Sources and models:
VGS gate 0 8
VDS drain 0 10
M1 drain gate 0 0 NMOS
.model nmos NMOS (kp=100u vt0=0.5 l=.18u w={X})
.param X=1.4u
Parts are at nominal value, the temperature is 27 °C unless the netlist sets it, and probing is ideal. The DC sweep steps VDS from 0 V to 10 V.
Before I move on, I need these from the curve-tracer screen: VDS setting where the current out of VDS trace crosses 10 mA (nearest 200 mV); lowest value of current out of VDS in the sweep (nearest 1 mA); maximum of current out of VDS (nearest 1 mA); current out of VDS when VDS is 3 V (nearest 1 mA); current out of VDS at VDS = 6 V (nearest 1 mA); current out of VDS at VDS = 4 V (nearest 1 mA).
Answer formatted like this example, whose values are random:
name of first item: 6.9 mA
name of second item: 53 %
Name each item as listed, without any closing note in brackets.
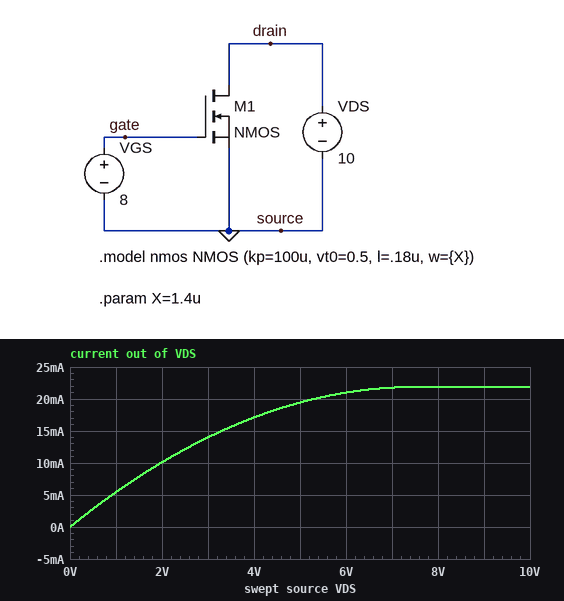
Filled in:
VDS setting where the current out of VDS trace crosses 10 mA: 2.0 V
lowest value of current out of VDS in the sweep: 0 A
maximum of current out of VDS: 22 mA
current out of VDS when VDS is 3 V: 14 mA
current out of VDS at VDS = 6 V: 21 mA
current out of VDS at VDS = 4 V: 17 mA
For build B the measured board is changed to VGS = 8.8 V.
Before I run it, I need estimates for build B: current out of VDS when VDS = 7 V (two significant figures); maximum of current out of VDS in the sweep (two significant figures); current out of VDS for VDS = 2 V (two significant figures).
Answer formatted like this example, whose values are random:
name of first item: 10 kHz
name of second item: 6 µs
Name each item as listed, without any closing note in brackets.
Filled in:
current out of VDS when VDS = 7 V: 26 mA
maximum of current out of VDS in the sweep: 27 mA
current out of VDS for VDS = 2 V: 11 mA
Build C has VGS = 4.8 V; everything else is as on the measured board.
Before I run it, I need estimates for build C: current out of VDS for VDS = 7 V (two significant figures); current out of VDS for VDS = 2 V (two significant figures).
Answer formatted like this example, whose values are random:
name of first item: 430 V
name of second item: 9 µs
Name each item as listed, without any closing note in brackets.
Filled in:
current out of VDS for VDS = 7 V: 7.2 mA
current out of VDS for VDS = 2 V: 5.1 mA
